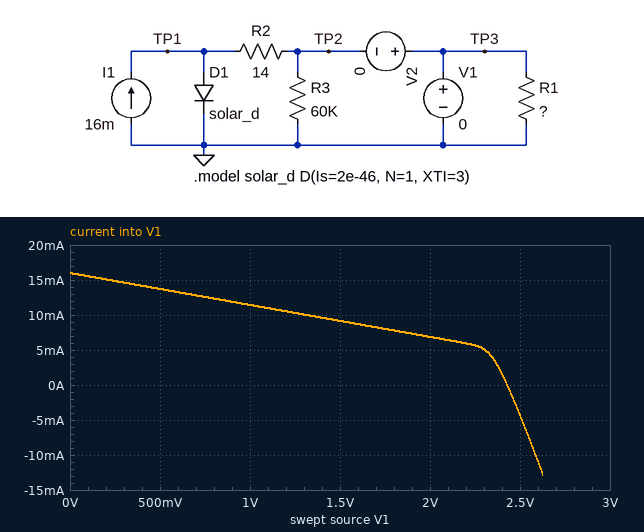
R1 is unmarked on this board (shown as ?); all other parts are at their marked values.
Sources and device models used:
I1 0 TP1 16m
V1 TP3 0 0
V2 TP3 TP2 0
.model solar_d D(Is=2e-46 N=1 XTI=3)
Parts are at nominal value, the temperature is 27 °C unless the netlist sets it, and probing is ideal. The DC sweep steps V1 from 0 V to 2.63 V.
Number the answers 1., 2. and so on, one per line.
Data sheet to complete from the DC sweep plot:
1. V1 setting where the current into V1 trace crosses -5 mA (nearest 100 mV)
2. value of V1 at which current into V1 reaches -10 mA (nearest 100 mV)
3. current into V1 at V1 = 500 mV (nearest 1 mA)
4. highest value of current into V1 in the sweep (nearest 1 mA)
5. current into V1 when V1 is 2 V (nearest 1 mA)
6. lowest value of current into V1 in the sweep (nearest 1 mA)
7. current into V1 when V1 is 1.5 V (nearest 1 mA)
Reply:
1. 2.5 V
2. 2.6 V
3. 14 mA
4. 16 mA
5. 7 mA
6. -13 mA
7. 9 mA
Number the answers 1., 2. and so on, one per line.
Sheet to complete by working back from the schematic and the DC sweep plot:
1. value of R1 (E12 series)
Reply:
1. 220 Ω
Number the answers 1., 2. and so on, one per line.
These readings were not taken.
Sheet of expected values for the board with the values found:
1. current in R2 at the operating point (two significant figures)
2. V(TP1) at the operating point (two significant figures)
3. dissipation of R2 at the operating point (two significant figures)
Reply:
1. 16 mA
2. 220 mV
3. 3.6 mW
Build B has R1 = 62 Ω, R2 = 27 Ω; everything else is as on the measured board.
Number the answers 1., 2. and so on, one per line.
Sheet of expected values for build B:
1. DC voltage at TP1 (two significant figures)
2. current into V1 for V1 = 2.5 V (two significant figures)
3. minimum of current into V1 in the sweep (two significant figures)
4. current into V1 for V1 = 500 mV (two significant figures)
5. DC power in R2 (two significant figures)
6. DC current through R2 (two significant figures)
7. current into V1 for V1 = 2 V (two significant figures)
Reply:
1. 430 mV
2. -36 mA
3. -43 mA
4. 7.9 mA
5. 6.9 mW
6. 16 mA
7. -16 mA
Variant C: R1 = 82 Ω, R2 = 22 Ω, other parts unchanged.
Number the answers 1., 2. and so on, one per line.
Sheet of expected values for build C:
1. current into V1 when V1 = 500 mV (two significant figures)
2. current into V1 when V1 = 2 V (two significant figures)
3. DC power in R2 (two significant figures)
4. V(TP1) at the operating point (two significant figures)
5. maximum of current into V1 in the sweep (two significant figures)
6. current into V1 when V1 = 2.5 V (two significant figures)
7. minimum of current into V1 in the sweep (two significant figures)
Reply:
1. 9.9 mA
2. -8.4 mA
3. 5.6 mW
4. 350 mV
5. 16 mA
6. -26 mA
7. -33 mA
